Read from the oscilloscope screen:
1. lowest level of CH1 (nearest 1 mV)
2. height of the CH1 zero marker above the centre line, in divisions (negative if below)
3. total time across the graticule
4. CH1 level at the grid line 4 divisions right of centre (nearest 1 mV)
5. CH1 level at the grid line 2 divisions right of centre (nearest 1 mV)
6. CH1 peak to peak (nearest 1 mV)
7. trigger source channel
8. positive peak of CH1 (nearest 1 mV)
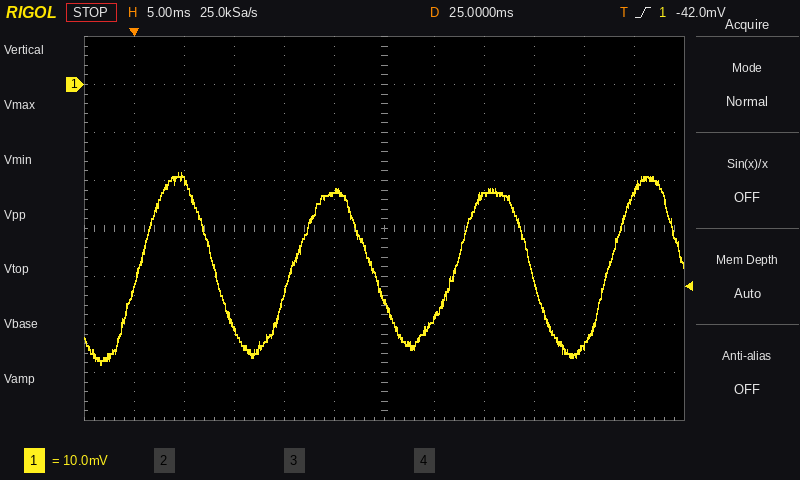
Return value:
-58 mV
+3.0 div
60 ms
-54 mV
-23 mV
40 mV
CH1
-18 mV
